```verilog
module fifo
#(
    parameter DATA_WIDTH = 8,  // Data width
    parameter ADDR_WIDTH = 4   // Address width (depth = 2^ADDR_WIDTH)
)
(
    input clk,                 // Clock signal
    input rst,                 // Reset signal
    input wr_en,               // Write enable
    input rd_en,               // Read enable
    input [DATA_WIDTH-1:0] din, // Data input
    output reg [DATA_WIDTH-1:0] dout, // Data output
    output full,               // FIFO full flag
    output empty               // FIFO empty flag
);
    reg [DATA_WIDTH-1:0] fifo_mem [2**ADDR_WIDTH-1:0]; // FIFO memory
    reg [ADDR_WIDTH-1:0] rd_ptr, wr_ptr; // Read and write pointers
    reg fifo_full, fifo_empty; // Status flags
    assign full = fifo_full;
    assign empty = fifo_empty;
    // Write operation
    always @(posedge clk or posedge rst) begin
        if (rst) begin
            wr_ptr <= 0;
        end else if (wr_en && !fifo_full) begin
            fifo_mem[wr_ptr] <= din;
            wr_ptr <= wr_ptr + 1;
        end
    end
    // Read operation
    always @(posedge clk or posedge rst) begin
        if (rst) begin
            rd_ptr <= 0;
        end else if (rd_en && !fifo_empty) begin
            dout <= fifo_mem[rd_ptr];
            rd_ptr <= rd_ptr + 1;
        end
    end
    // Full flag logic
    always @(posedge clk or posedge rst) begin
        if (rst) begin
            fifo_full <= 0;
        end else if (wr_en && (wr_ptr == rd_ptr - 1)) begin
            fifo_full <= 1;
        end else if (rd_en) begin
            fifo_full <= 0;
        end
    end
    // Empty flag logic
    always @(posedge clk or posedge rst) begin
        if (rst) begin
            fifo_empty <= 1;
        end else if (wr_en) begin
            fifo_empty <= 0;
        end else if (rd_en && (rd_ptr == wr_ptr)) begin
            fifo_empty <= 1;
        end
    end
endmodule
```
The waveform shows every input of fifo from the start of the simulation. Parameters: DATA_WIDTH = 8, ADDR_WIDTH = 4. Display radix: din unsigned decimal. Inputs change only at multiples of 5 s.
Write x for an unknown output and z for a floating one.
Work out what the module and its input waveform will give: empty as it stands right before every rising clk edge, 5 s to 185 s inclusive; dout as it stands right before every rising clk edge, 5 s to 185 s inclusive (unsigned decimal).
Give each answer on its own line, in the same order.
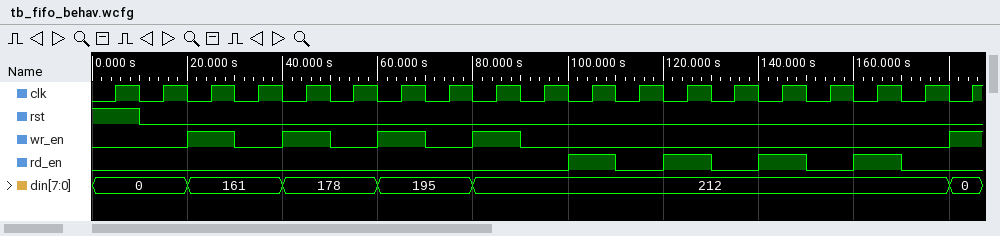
1 1 1 0 0 0 0 0 0 0 0 0 0 0 0 0 0 0 0
x, x, x, x, x, x, x, x, x, x, x, 161, 161, 178, 178, 195, 195, 212, 212
